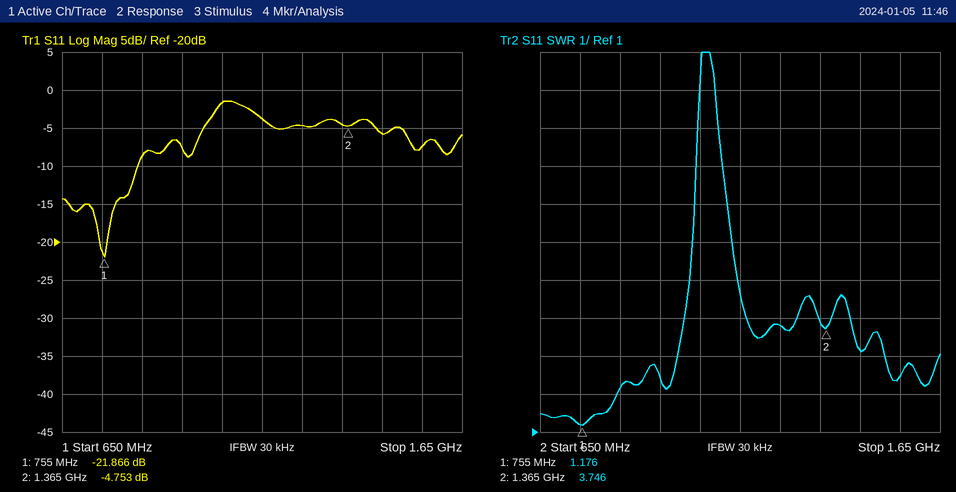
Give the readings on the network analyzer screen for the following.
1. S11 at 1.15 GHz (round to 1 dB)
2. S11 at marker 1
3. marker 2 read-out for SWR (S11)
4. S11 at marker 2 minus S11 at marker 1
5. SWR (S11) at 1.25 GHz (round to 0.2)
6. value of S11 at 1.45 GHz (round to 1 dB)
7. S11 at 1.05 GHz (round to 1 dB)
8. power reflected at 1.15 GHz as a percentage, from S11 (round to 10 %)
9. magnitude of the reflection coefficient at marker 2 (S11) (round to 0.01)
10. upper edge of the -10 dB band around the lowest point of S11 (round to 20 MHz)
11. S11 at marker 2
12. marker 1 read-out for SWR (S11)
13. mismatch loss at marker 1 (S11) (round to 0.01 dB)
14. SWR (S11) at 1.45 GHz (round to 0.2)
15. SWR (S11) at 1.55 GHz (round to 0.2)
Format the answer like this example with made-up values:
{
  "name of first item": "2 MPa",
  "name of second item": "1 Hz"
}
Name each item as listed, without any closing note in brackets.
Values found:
{
  "S11 at 1.15 GHz": "-4 dB",
  "S11 at marker 1": "-21.866 dB",
  "marker 2 read-out for SWR": "3.746",
  "S11 at marker 2 minus S11 at marker 1": "17.113 dB",
  "SWR (S11) at 1.25 GHz": "3.8",
  "value of S11 at 1.45 GHz": "-6 dB",
  "S11 at 1.05 GHz": "-2 dB",
  "power reflected at 1.15 GHz as a percentage, from S11": "40 %",
  "magnitude of the reflection coefficient at marker 2 (S11)": "0.58",
  "upper edge of the -10 dB band around the lowest point of S11": "840 MHz",
  "S11 at marker 2": "-4.753 dB",
  "marker 1 read-out for SWR": "1.176",
  "mismatch loss at marker 1 (S11)": "0.03 dB",
  "SWR (S11) at 1.45 GHz": "3.2",
  "SWR (S11) at 1.55 GHz": "2.4"
}
